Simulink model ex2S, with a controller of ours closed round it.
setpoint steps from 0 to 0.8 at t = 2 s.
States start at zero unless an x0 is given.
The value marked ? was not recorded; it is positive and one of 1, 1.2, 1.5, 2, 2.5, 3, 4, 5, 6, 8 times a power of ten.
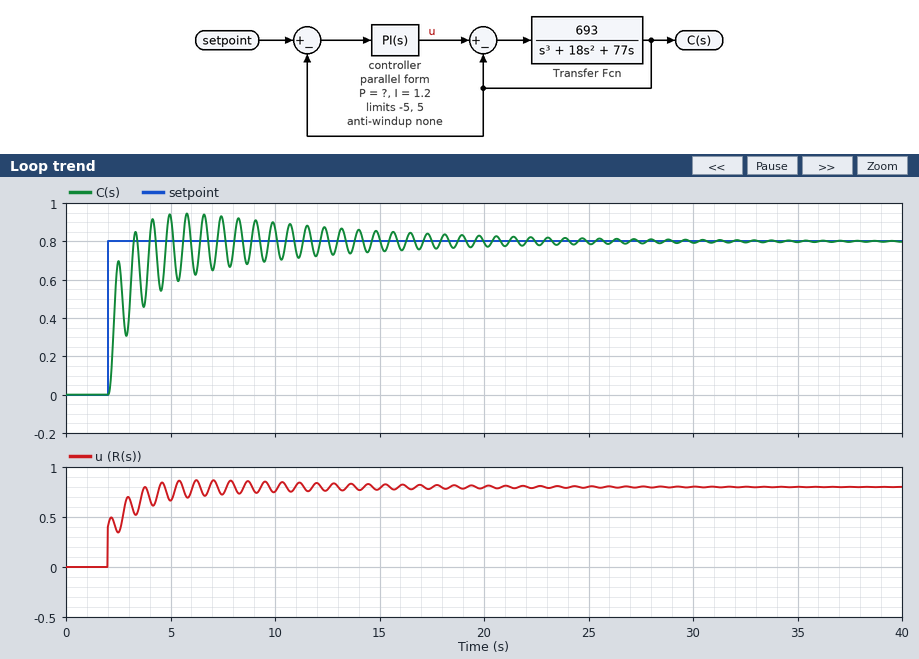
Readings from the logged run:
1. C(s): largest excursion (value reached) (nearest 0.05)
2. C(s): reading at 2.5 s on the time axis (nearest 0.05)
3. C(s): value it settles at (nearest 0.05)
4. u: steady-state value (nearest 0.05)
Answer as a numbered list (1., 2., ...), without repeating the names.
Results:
1. 0.95
2. 0.70
3. 0.80
4. 0.80
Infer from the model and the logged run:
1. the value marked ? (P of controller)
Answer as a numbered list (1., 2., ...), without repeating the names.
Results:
1. 0.5
